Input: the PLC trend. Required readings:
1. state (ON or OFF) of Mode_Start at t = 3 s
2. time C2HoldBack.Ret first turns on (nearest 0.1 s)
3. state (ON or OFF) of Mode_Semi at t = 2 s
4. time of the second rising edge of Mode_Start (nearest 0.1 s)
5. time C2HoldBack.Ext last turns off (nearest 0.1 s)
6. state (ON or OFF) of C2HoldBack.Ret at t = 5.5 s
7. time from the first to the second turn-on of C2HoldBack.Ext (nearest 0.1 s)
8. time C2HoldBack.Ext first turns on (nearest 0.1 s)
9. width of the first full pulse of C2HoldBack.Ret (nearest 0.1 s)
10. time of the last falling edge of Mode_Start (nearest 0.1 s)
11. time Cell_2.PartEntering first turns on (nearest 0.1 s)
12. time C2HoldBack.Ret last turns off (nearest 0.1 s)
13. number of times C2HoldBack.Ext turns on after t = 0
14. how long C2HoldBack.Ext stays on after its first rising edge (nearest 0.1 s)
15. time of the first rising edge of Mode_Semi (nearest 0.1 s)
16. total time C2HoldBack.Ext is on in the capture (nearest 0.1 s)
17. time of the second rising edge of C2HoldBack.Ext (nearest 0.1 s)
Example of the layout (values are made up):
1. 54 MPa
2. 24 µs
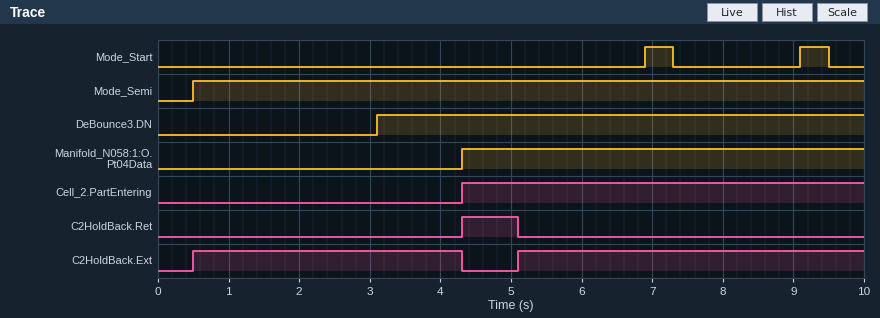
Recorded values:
1. OFF
2. 4.3 s
3. ON
4. 9.1 s
5. 4.3 s
6. OFF
7. 4.6 s
8. 0.5 s
9. 0.8 s
10. 9.5 s
11. 4.3 s
12. 5.1 s
13. 2
14. 3.8 s
15. 0.5 s
16. 8.7 s
17. 5.1 s
